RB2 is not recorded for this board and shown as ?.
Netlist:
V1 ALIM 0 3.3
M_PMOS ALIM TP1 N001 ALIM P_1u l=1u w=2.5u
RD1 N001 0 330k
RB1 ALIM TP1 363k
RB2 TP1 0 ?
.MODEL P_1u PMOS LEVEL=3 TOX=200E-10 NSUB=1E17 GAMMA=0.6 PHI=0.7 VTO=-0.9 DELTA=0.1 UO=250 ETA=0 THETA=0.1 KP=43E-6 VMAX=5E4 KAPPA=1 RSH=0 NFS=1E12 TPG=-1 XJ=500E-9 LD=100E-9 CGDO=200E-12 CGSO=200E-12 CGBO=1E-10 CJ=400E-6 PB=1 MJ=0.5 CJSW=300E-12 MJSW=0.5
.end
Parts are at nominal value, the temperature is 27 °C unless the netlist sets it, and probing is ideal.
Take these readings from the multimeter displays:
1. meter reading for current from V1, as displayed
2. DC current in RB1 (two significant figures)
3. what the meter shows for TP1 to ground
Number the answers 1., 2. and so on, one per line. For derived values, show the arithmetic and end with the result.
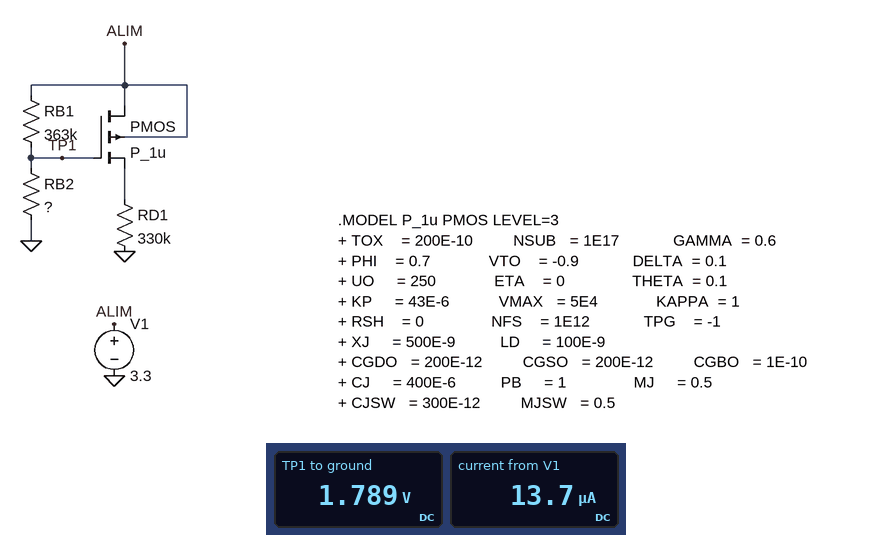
1. 13.7 µA
2. (3.3 V - 1.789 V) / 363 kΩ = 4.2 µA
3. 1.789 V
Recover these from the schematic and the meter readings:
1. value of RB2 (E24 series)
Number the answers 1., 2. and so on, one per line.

1. 430 kΩ
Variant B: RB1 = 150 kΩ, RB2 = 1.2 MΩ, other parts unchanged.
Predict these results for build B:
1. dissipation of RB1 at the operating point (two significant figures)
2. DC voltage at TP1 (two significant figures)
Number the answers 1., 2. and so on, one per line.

1. 900 nW
2. 2.9 V
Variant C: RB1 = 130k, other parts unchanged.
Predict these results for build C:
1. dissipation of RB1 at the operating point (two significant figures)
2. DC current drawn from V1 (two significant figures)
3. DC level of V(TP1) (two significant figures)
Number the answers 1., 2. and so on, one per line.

1. 4.5 µW
2. 5.9 µA
3. 2.5 V
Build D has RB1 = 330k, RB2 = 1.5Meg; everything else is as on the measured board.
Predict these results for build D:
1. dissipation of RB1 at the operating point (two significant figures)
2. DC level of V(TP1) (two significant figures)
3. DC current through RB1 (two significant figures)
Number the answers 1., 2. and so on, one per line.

1. 1.1 µW
2. 2.7 V
3. 1.8 µA
